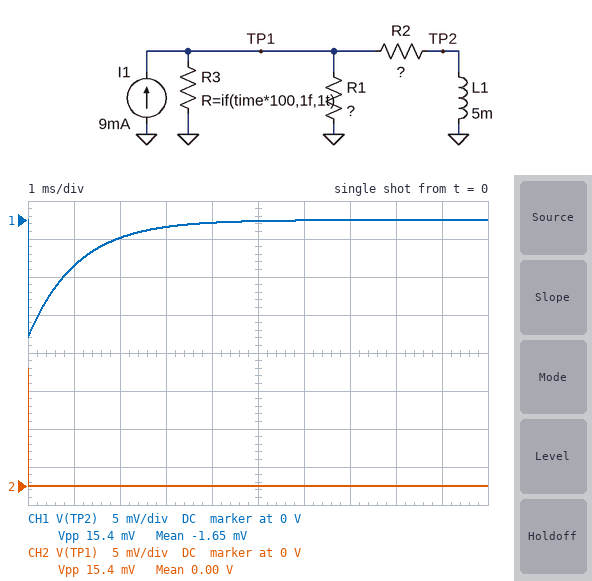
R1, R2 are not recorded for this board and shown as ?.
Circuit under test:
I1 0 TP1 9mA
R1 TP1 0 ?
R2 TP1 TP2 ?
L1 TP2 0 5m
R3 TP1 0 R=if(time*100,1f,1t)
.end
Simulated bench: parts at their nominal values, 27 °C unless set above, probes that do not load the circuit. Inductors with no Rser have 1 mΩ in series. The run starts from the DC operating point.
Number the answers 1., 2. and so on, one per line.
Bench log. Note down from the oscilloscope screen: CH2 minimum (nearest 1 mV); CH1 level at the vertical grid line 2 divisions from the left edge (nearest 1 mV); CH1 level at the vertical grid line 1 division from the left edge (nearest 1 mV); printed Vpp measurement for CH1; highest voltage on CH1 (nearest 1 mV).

1. 0 V
2. -2 mV
3. -6 mV
4. 15.4 mV
5. 0 V
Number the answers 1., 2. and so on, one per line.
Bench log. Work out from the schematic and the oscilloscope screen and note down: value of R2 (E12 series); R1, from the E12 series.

1. 4.7 Ω
2. 2.7 Ω
